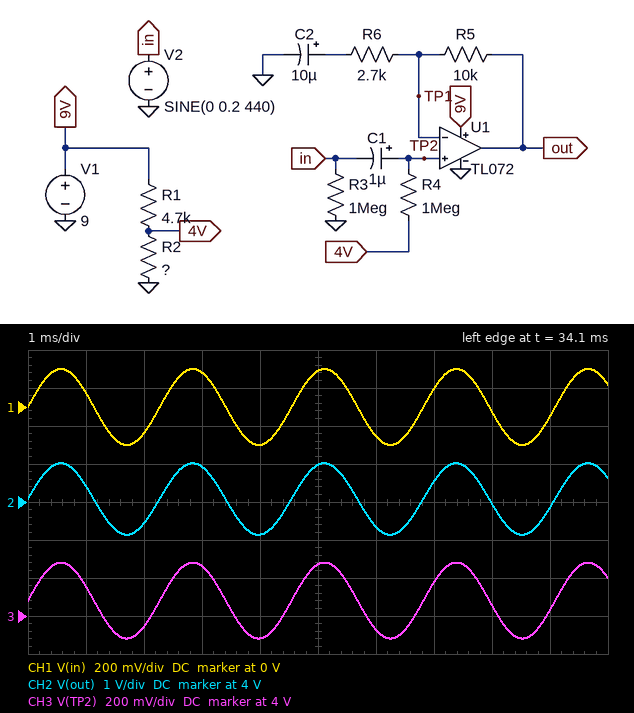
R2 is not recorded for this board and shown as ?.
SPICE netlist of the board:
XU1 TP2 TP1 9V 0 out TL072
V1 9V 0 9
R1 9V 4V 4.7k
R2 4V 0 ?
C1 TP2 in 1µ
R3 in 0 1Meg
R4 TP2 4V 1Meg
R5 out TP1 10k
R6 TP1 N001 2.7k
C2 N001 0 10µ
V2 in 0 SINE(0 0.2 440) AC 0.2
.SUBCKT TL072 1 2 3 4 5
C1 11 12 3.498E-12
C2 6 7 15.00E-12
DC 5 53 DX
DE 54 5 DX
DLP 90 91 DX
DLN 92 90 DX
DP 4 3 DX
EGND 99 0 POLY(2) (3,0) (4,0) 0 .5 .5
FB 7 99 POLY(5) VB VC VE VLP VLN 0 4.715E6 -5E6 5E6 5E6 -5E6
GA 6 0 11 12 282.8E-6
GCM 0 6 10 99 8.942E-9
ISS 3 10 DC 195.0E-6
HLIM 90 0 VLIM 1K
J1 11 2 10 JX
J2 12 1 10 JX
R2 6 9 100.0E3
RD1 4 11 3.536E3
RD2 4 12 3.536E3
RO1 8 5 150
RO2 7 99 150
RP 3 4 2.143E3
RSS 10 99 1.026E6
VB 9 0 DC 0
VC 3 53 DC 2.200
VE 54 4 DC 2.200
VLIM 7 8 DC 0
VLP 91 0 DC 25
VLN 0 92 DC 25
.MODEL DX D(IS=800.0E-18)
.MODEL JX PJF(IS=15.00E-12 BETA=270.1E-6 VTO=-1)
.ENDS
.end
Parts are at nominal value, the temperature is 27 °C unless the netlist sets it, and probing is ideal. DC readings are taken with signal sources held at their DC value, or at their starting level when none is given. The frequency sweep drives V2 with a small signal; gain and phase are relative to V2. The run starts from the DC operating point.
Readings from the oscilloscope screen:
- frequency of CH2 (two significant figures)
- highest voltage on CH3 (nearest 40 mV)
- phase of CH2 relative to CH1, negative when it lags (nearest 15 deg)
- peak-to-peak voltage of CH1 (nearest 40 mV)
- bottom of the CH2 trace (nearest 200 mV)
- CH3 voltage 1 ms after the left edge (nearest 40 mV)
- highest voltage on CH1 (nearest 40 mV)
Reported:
440 Hz
4.28 V
0 deg
400 mV
3.2 V
4.16 V
200 mV
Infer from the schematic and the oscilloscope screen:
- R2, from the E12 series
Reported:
3.9 kΩ
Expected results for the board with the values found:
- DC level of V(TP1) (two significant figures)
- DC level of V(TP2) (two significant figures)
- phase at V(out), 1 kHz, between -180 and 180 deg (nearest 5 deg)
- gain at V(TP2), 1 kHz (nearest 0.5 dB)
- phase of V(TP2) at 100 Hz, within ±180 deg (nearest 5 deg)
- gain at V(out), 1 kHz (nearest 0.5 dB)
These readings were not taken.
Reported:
4.1 V
4.1 V
0 deg
0 dB
0 deg
13.5 dB
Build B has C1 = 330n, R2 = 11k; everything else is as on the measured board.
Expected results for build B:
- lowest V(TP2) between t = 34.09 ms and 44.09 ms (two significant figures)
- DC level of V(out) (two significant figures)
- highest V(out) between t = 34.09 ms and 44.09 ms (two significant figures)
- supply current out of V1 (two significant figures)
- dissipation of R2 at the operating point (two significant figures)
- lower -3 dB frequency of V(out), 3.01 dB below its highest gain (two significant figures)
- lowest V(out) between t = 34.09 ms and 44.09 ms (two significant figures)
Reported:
6.1 V
6.3 V
7.2 V
5.0 mA
3.6 mW
5.7 Hz
5.4 V
